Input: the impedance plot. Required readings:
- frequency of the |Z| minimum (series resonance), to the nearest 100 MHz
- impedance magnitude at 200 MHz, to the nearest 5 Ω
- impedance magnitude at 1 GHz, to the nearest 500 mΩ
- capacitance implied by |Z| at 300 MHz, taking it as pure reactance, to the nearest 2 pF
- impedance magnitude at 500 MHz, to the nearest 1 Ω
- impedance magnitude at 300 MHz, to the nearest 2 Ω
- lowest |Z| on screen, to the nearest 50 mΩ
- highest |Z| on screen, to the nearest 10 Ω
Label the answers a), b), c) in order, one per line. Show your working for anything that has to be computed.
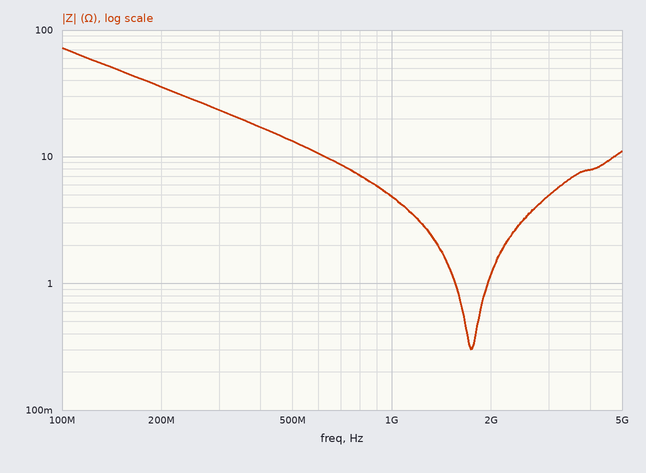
a) 1.7 GHz
b) 35 Ω
c) 5.0 Ω
d) C = 1/(2π × 300 MHz × 24 Ω) ≈ 22 pF
e) 13 Ω
f) 24 Ω
g) 300 mΩ
h) 70 Ω
